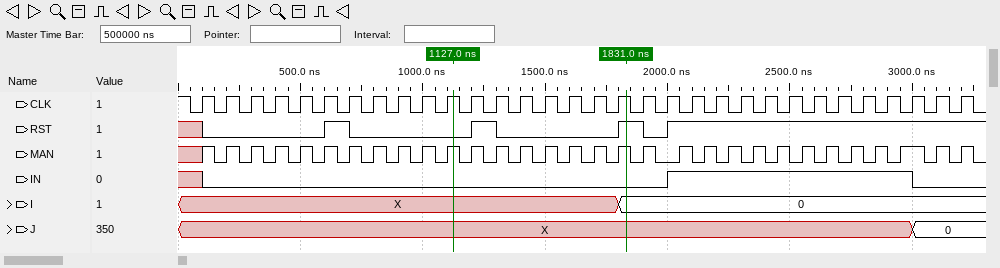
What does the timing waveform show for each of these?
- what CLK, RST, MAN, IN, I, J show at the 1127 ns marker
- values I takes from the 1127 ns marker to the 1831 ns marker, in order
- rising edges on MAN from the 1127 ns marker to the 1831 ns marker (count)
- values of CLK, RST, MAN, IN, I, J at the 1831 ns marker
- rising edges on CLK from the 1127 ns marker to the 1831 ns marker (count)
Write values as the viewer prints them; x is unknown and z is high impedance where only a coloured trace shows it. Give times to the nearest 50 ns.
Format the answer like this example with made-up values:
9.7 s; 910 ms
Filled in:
CLK=1, RST=0, MAN=1, IN=0, I=X, J=X; X, 0; 7; CLK=1, RST=1, MAN=1, IN=0, I=0, J=X; 7
